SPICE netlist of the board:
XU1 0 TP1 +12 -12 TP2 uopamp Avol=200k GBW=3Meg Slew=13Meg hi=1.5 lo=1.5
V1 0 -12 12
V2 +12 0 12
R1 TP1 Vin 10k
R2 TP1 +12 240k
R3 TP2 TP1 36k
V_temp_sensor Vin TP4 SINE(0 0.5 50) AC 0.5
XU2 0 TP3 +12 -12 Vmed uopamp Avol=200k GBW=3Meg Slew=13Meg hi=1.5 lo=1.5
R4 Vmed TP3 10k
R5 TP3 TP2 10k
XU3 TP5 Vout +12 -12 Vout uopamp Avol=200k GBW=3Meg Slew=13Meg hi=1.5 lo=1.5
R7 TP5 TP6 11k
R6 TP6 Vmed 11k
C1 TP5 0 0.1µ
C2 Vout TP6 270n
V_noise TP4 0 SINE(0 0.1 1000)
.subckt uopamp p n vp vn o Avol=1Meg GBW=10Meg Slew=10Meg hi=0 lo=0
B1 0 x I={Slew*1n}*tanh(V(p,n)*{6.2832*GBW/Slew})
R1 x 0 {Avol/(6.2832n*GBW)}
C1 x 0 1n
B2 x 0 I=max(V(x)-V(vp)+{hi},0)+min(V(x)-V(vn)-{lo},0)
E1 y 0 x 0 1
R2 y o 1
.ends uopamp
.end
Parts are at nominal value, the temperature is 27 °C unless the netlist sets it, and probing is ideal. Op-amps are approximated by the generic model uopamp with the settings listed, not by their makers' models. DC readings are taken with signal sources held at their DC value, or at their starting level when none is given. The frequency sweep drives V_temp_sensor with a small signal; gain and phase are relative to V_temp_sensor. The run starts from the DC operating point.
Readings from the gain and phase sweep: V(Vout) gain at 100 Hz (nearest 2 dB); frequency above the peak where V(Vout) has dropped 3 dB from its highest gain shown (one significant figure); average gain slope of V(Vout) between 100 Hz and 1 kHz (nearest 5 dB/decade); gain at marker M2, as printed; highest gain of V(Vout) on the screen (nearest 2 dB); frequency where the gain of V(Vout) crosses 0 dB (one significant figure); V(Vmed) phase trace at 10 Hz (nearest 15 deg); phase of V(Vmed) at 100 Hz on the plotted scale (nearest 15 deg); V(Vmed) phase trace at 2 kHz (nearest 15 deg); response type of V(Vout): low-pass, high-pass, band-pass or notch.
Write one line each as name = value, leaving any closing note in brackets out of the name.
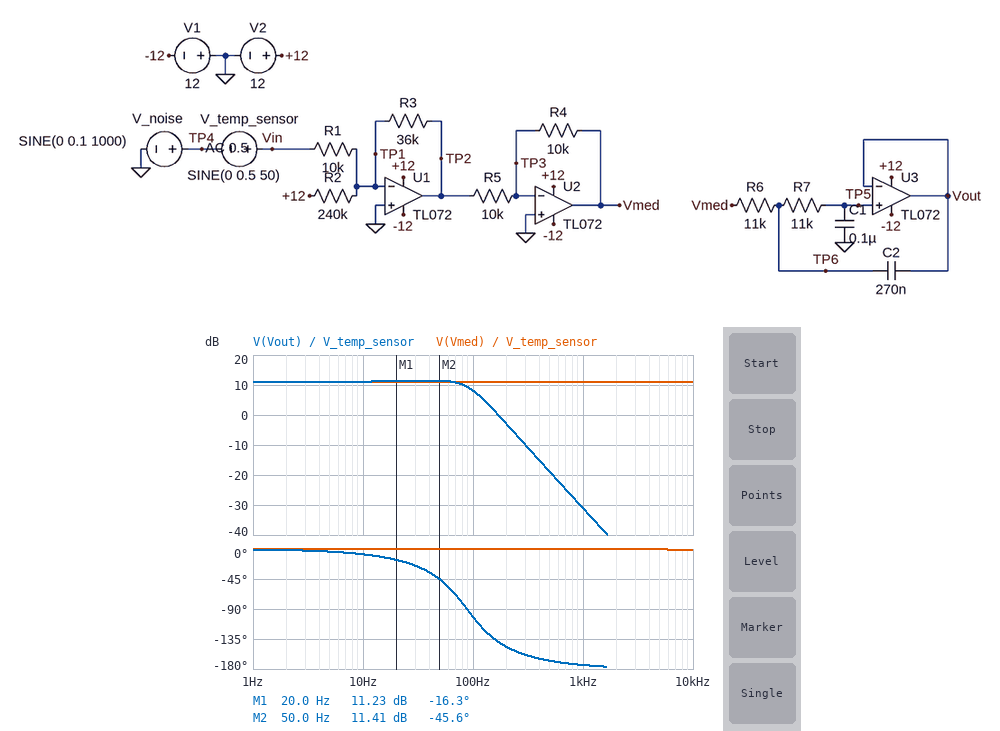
V(Vout) gain at 100 Hz = 8 dB
frequency above the peak where V(Vout) has dropped 3 dB from its highest gain shown = 100 Hz
average gain slope of V(Vout) between 100 Hz and 1 kHz = -40 dB/decade
gain at marker M2, as printed = 11.41 dB
highest gain of V(Vout) on the screen = 12 dB
frequency where the gain of V(Vout) crosses 0 dB = 200 Hz
V(Vmed) phase trace at 10 Hz = 0 deg
phase of V(Vmed) at 100 Hz on the plotted scale = 0 deg
V(Vmed) phase trace at 2 kHz = 0 deg
response type of V(Vout): low-pass, high-pass, band-pass or notch = low-pass
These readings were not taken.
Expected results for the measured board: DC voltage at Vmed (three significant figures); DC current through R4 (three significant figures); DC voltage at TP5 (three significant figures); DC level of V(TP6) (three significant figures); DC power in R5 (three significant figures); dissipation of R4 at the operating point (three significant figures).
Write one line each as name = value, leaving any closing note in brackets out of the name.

DC voltage at Vmed = 1.80 V
DC current through R4 = 180 µA
DC voltage at TP5 = 1.80 V
DC level of V(TP6) = 1.80 V
DC power in R5 = 324 µW
dissipation of R4 at the operating point = 324 µW
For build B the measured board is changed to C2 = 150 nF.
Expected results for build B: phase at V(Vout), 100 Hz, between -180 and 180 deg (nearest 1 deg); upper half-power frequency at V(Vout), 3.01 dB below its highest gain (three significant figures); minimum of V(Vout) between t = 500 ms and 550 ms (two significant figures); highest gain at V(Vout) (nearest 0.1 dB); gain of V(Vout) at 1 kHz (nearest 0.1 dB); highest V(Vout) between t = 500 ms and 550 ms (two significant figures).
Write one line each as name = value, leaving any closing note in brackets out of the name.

phase at V(Vout), 100 Hz, between -180 and 180 deg = -78 deg
upper half-power frequency at V(Vout), 3.01 dB below its highest gain = 100 Hz
minimum of V(Vout) between t = 500 ms and 550 ms = 120 mV
highest gain at V(Vout) = 11.1 dB
gain of V(Vout) at 1 kHz = -26.0 dB
highest V(Vout) between t = 500 ms and 550 ms = 3.5 V
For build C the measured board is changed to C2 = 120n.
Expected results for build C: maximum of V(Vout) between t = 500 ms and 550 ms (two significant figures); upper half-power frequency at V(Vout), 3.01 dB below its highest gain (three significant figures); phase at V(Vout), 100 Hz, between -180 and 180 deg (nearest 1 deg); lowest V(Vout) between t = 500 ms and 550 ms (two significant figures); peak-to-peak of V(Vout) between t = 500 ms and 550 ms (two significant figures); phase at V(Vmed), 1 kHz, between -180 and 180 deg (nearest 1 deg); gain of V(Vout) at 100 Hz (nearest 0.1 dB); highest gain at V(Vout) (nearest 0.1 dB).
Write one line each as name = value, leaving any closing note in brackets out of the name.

maximum of V(Vout) between t = 500 ms and 550 ms = 3.4 V
upper half-power frequency at V(Vout), 3.01 dB below its highest gain = 96.6 Hz
phase at V(Vout), 100 Hz, between -180 and 180 deg = -73 deg
lowest V(Vout) between t = 500 ms and 550 ms = 160 mV
peak-to-peak of V(Vout) between t = 500 ms and 550 ms = 3.3 V
phase at V(Vmed), 1 kHz, between -180 and 180 deg = 0 deg
gain of V(Vout) at 100 Hz = 7.9 dB
highest gain at V(Vout) = 11.1 dB
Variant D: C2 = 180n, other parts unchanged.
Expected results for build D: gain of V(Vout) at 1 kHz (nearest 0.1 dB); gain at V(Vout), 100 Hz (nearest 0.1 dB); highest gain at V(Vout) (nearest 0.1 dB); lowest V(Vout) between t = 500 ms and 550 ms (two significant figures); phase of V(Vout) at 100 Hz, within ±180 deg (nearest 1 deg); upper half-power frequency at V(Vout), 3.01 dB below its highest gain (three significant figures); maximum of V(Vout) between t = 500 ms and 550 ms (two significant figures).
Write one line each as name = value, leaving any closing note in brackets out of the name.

gain of V(Vout) at 1 kHz = -27.6 dB
gain at V(Vout), 100 Hz = 8.3 dB
highest gain at V(Vout) = 11.1 dB
lowest V(Vout) between t = 500 ms and 550 ms = 75 mV
phase of V(Vout) at 100 Hz, within ±180 deg = -84 deg
upper half-power frequency at V(Vout), 3.01 dB below its highest gain = 102 Hz
maximum of V(Vout) between t = 500 ms and 550 ms = 3.5 V
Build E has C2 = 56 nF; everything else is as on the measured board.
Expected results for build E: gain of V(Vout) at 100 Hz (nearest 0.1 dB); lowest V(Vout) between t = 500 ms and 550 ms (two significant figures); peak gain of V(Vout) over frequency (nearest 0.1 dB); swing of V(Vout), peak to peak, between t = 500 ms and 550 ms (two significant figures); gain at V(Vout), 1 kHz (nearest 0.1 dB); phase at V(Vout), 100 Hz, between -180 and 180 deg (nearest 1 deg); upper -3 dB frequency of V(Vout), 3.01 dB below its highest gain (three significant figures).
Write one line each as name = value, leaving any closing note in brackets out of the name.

gain of V(Vout) at 100 Hz = 7.2 dB
lowest V(Vout) between t = 500 ms and 550 ms = 240 mV
peak gain of V(Vout) over frequency = 11.1 dB
swing of V(Vout), peak to peak, between t = 500 ms and 550 ms = 3.1 V
gain at V(Vout), 1 kHz = -18.2 dB
phase at V(Vout), 100 Hz, between -180 and 180 deg = -62 deg
upper -3 dB frequency of V(Vout), 3.01 dB below its highest gain = 83.7 Hz
